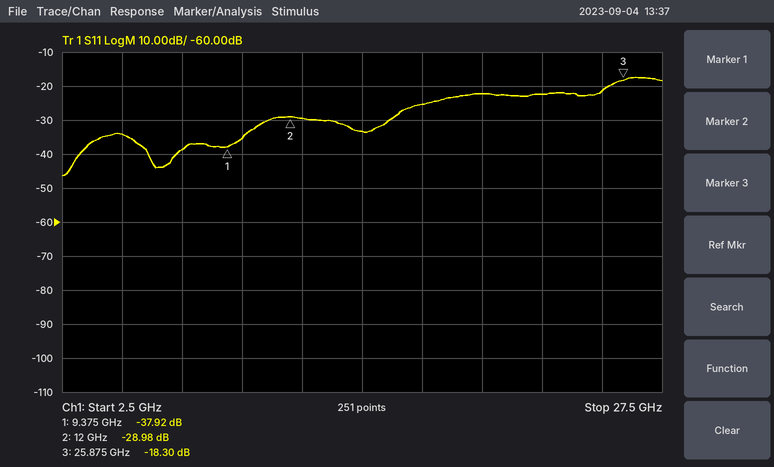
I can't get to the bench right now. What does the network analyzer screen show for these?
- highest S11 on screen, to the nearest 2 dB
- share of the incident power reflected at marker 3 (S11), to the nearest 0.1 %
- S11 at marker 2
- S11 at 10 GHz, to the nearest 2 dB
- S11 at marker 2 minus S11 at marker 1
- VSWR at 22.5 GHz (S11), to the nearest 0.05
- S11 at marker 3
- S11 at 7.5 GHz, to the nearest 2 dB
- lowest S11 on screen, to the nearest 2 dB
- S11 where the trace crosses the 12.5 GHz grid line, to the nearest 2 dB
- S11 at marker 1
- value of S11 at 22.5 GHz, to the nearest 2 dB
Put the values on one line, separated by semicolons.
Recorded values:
-18 dB; 1.5 %; -28.98 dB; -36 dB; 8.94 dB; 1.15; -18.30 dB; -38 dB; -46 dB; -30 dB; -37.92 dB; -22 dB
